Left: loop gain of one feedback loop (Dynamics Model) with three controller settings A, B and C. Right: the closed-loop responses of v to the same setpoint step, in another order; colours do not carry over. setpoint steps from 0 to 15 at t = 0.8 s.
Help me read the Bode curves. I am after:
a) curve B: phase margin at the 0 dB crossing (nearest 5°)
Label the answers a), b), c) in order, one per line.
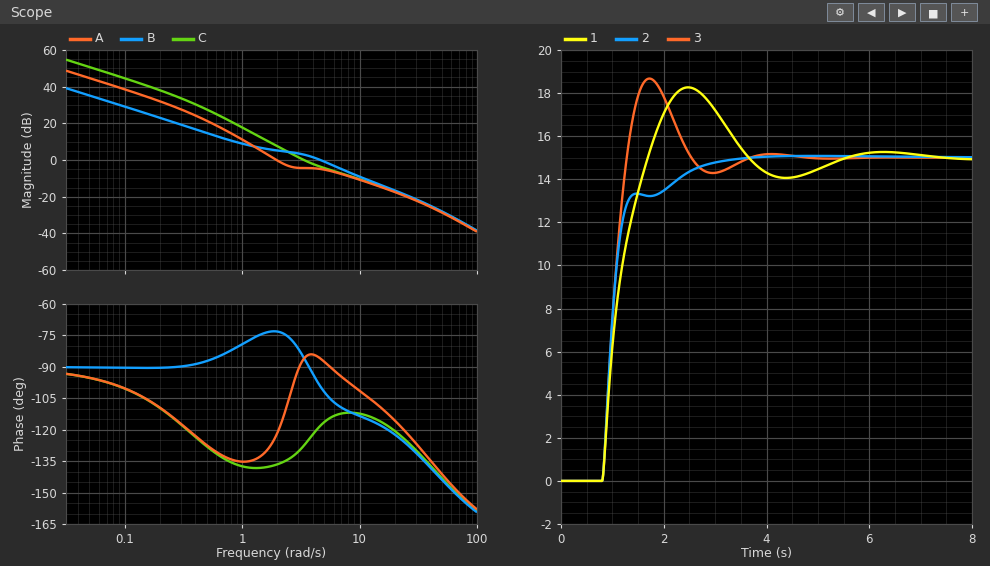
a) 80°
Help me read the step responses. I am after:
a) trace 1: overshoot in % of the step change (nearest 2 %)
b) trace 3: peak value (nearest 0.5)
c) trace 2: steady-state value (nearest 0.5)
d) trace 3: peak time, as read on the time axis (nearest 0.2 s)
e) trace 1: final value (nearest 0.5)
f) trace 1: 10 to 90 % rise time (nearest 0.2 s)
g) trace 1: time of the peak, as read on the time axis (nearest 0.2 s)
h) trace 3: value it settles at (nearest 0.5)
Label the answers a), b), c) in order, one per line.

a) 22 %
b) 18.5
c) 15.0
d) 1.8 s
e) 15.0
f) 0.6 s
g) 2.4 s
h) 15.0
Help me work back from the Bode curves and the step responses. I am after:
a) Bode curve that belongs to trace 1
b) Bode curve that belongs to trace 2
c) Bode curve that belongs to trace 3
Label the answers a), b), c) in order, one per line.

a) A
b) B
c) C
